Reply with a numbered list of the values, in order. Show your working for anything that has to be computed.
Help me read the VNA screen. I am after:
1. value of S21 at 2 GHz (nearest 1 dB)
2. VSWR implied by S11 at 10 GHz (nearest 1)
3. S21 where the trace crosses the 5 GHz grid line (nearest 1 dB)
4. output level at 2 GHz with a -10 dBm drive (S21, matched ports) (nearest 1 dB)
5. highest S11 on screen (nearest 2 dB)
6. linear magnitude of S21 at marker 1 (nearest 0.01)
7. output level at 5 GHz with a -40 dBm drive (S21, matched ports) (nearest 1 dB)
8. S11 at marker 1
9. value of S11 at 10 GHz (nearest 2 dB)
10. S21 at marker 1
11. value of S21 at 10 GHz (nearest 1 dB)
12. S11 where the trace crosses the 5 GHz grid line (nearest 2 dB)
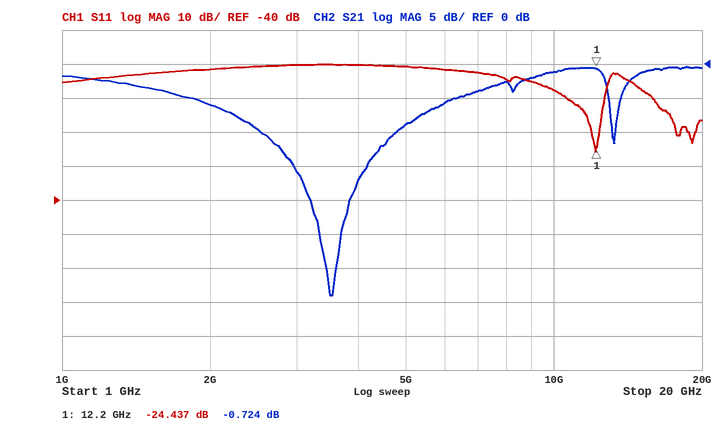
1. -6 dB
2. |Γ| = 10^(-8/20) = 0.3981; VSWR = (1 + 0.3981)/(1 − 0.3981) ≈ 2
3. -9 dB
4. -10 dBm + (-6 dB) = -16 dBm
5. 0 dB
6. 10^(-0.724/20) ≈ 0.92
7. -40 dBm + (-9 dB) = -49 dBm
8. -24.437 dB
9. -8 dB
10. -0.724 dB
11. -1 dB
12. 0 dB
